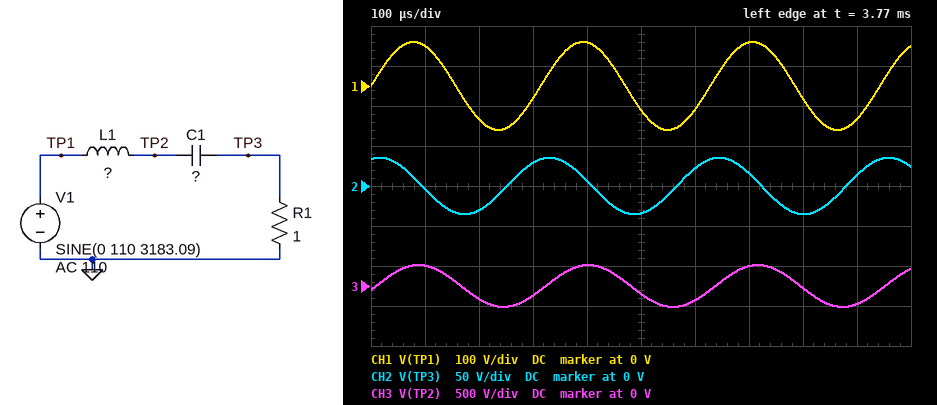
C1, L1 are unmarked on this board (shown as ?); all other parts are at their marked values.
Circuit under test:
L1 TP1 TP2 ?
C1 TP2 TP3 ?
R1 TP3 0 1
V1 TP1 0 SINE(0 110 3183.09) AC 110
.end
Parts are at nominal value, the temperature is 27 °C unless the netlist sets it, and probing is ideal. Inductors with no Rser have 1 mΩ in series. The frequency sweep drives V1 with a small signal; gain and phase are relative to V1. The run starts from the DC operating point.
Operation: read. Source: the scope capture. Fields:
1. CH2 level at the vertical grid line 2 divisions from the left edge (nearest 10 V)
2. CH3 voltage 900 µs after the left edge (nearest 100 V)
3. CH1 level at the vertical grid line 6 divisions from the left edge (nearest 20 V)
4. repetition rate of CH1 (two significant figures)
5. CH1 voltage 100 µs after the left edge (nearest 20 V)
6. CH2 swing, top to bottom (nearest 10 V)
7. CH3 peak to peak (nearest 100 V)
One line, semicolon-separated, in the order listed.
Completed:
-30 V; -200 V; -60 V; 3.2 kHz; 100 V; 70 V; 500 V
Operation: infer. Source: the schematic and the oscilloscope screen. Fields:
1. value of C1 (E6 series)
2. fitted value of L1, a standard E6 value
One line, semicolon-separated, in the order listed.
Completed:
6.8 µF; 220 µH
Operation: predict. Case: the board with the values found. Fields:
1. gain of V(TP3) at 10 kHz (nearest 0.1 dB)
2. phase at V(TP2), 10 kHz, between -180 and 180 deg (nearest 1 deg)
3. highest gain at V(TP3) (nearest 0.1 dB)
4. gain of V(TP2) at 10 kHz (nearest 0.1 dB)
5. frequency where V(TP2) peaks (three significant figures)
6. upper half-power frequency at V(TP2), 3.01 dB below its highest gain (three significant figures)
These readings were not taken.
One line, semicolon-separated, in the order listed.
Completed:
-21.2 dB; -152 deg; 0 dB; -13.1 dB; 4.08 kHz; 4.43 kHz
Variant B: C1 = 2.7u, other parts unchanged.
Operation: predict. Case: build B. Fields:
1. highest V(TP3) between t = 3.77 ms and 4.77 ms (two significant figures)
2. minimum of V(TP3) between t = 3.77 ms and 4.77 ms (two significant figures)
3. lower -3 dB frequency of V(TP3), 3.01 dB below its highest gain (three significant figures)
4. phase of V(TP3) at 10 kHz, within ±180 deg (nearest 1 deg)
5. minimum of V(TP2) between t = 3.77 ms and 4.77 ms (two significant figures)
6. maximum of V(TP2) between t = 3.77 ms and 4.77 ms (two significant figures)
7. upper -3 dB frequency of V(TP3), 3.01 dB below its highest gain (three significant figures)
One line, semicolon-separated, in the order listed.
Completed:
7.8 V; -7.8 V; 6.18 kHz; -83 deg; -140 V; 140 V; 6.90 kHz
